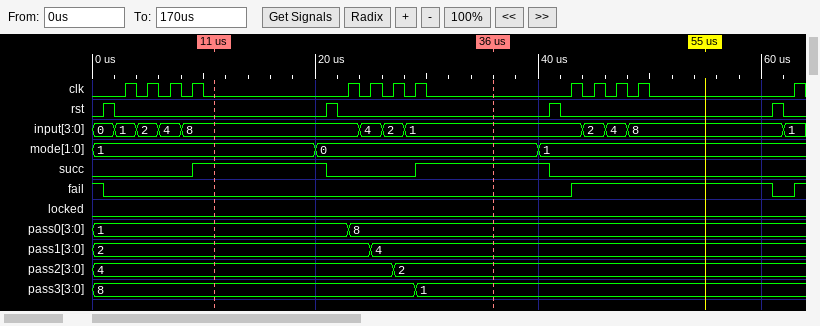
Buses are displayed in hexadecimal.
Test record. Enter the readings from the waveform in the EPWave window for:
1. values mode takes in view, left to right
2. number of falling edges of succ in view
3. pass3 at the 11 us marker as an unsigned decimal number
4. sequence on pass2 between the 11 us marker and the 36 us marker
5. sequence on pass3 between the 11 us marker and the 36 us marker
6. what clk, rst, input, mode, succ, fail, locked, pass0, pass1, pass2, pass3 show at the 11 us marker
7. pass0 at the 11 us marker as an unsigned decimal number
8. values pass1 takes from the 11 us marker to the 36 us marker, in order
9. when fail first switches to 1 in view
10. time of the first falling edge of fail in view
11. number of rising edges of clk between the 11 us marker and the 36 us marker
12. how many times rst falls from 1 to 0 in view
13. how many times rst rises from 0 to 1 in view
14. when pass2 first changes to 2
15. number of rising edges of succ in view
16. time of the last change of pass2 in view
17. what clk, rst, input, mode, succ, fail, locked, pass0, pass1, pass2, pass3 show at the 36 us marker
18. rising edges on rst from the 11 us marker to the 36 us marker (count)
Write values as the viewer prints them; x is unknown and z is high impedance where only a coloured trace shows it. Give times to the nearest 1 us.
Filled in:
1, 0, 1
2
8
4, 2
8, 1
clk=0, rst=0, input=8, mode=1, succ=1, fail=0, locked=0, pass0=1, pass1=2, pass2=4, pass3=8
1
2, 4
43 us
1 us
4
4
4
27 us
2
27 us
clk=0, rst=0, input=1, mode=0, succ=1, fail=0, locked=0, pass0=8, pass1=4, pass2=2, pass3=1
1
